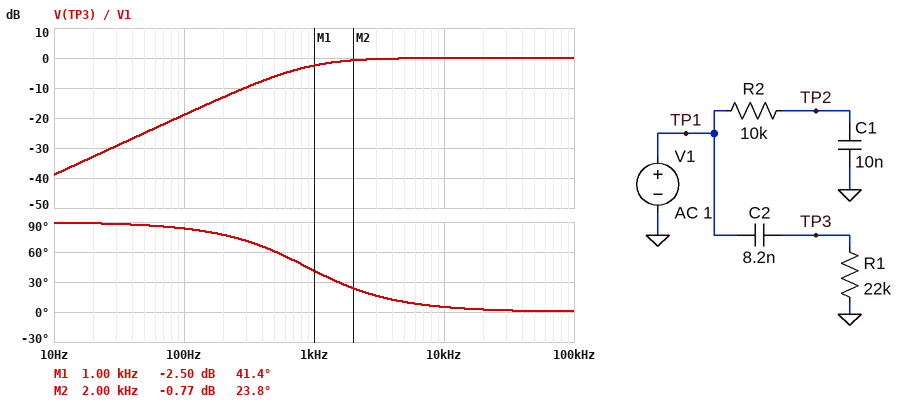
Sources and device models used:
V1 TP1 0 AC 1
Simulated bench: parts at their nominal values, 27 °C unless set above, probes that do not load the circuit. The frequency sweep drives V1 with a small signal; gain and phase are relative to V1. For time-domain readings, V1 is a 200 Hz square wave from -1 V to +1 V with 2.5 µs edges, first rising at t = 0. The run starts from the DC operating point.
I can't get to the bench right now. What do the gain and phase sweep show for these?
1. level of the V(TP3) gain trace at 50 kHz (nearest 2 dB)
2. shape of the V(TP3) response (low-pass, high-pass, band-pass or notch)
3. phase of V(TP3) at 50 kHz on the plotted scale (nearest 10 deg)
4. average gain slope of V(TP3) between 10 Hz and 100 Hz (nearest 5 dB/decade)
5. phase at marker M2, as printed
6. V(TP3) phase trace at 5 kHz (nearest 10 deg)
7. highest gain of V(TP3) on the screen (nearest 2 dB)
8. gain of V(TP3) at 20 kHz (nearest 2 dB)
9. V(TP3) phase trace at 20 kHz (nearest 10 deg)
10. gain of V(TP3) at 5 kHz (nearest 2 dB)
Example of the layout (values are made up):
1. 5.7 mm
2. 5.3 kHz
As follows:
1. 0 dB
2. high-pass
3. 0 deg
4. 20 dB/decade
5. 23.8 deg
6. 10 deg
7. 0 dB
8. 0 dB
9. 0 deg
10. 0 dB
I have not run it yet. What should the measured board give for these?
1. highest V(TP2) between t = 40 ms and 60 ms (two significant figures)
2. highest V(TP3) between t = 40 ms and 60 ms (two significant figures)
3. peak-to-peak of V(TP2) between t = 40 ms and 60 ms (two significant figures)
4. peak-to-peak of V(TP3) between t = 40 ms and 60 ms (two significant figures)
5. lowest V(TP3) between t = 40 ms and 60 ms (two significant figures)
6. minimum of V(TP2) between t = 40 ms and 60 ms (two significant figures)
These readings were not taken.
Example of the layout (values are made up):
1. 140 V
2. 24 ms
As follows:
1. 1.0 V
2. 2.0 V
3. 2.0 V
4. 4.0 V
5. -2.0 V
6. -1.0 V
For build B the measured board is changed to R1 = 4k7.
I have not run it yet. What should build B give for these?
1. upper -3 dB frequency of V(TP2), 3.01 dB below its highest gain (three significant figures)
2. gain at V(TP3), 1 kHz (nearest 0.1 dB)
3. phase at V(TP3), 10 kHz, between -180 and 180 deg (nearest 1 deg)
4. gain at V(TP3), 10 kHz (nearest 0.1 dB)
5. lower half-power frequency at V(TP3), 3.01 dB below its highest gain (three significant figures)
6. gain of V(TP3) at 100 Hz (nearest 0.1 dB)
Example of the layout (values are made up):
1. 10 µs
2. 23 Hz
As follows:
1. 1.59 kHz
2. -12.6 dB
3. 22 deg
4. -0.7 dB
5. 4.13 kHz
6. -32.3 dB
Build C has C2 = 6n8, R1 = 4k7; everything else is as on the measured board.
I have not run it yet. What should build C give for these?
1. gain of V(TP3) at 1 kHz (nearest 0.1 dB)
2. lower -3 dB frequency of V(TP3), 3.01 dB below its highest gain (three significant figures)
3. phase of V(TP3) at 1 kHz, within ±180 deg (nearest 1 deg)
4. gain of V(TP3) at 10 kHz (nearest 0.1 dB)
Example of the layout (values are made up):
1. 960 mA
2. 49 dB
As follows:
1. -14.1 dB
2. 4.98 kHz
3. 79 deg
4. -1.0 dB
